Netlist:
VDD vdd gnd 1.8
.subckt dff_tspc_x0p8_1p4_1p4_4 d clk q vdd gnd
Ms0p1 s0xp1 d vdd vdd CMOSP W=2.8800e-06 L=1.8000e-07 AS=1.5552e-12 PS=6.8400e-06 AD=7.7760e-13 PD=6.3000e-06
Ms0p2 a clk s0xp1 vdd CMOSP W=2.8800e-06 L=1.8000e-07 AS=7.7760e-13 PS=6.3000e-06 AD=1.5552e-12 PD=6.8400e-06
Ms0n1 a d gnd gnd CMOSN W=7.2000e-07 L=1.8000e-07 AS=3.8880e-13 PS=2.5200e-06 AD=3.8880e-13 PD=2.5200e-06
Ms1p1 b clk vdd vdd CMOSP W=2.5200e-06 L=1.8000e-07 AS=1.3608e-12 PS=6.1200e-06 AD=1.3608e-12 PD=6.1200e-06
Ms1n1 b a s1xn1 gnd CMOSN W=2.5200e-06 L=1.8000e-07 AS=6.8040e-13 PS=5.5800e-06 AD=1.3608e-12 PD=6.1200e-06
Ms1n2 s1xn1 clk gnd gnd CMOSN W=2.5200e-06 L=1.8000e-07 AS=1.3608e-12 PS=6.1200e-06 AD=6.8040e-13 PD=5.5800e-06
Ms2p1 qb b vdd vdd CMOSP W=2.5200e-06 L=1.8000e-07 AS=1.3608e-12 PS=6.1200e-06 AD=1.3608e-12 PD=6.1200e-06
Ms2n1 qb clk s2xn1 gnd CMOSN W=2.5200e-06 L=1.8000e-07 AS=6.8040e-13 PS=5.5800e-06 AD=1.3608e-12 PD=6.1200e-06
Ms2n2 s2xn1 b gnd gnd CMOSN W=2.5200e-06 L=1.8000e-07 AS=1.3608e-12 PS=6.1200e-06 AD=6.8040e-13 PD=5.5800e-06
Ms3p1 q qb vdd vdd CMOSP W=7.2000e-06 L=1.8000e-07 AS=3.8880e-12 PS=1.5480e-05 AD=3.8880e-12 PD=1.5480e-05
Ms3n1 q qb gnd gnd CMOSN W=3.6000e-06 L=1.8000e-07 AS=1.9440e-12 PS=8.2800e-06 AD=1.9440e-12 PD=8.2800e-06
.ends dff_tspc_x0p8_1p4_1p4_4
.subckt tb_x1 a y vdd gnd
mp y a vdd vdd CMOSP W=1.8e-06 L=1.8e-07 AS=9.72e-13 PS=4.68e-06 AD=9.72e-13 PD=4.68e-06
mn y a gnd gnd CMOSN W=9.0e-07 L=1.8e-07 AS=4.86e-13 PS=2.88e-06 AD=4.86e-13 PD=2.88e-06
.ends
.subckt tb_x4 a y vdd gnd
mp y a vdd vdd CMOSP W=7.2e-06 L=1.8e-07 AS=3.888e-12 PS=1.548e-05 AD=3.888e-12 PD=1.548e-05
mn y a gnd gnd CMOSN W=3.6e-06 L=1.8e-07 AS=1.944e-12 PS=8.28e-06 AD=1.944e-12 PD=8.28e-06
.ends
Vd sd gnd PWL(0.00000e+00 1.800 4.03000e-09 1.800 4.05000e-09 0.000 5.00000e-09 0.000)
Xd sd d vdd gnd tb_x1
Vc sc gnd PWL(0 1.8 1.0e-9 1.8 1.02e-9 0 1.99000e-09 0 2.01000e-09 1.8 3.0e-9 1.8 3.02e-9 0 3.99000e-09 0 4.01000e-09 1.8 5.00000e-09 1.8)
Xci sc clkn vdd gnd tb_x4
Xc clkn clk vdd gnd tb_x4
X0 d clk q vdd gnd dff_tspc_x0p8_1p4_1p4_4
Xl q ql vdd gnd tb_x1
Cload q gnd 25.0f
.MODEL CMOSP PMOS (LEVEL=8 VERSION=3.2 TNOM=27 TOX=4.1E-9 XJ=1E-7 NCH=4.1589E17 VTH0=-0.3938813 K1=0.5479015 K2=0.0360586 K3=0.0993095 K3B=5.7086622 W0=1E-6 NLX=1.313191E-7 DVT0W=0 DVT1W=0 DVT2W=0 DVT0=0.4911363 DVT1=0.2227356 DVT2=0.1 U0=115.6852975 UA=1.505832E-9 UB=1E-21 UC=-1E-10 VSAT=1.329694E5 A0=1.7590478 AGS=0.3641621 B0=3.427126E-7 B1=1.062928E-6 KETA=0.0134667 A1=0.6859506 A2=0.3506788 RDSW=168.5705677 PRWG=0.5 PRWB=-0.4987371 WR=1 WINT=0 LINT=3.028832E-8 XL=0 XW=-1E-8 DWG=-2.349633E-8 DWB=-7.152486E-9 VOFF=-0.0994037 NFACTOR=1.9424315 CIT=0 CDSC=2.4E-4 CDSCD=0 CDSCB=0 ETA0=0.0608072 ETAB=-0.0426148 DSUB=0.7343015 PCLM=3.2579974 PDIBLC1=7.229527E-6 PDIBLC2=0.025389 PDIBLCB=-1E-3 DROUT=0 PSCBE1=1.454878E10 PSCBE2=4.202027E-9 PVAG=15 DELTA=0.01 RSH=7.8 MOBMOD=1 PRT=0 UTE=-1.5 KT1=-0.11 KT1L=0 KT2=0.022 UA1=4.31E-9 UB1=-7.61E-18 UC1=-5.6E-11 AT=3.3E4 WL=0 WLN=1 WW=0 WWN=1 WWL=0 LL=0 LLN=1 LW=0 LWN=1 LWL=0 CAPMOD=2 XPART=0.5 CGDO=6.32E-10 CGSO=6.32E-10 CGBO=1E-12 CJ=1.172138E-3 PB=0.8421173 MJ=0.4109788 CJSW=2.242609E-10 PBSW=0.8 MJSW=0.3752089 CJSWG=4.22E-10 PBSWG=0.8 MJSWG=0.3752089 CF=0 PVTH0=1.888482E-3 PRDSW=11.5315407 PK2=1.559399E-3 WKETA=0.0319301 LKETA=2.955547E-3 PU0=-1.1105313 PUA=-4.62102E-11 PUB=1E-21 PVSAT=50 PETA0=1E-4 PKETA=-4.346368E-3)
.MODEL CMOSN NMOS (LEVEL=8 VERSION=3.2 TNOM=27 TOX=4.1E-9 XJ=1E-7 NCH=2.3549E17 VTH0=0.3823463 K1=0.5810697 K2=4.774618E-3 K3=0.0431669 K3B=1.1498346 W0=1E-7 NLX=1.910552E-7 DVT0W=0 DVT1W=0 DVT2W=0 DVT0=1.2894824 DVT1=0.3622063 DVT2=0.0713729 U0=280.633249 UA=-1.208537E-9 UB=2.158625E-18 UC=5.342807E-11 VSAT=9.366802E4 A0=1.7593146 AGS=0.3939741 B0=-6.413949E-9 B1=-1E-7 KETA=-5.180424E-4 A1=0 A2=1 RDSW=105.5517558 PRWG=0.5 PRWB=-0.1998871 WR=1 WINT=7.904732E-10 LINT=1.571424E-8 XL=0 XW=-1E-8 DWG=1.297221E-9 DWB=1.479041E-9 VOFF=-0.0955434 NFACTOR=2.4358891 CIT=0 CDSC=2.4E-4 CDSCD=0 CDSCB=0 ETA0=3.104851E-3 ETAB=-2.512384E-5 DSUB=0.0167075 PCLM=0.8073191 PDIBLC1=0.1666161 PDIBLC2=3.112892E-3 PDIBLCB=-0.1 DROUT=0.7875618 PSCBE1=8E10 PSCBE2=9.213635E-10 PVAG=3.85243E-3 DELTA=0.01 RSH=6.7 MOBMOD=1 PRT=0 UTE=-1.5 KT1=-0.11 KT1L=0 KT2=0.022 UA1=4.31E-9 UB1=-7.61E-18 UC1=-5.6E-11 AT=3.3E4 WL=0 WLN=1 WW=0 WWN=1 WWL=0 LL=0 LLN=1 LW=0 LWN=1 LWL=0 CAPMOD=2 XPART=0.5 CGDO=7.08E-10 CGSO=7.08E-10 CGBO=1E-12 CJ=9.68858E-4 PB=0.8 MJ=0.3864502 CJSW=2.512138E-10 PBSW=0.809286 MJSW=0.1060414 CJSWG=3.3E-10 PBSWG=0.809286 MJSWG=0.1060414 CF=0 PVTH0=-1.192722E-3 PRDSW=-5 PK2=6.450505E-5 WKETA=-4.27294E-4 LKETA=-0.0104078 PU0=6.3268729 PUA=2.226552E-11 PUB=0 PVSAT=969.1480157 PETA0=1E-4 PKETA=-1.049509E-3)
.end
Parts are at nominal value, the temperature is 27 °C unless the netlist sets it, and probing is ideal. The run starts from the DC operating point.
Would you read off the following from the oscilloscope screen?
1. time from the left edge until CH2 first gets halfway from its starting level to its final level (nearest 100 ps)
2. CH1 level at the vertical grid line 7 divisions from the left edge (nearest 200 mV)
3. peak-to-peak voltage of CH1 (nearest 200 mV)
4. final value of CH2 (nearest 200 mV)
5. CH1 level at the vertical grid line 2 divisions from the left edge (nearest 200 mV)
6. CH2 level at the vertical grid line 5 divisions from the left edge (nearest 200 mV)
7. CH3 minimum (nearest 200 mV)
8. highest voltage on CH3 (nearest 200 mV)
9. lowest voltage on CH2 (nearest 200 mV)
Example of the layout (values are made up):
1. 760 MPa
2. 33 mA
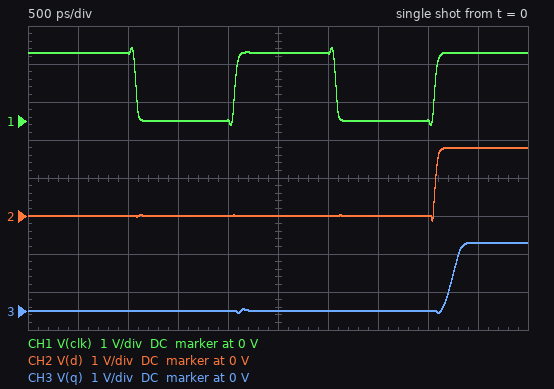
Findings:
1. 4.1 ns
2. 0 V
3. 2.0 V
4. 1.8 V
5. 1.8 V
6. 0 V
7. 0 V
8. 1.8 V
9. -200 mV
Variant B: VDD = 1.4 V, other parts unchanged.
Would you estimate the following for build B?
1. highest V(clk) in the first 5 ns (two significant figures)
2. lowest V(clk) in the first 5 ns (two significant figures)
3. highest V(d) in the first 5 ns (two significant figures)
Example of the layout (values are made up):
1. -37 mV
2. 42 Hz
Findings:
1. 1.5 V
2. -140 mV
3. 1.4 V
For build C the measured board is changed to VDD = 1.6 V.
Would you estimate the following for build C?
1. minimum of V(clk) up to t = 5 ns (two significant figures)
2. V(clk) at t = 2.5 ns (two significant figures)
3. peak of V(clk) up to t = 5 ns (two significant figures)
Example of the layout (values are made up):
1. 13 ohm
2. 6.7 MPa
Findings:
1. -120 mV
2. 1.6 V
3. 1.7 V
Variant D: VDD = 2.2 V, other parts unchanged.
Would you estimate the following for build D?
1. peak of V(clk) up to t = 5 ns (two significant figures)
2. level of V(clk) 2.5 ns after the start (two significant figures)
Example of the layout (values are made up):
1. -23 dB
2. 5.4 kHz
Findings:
1. 2.3 V
2. 2.2 V
